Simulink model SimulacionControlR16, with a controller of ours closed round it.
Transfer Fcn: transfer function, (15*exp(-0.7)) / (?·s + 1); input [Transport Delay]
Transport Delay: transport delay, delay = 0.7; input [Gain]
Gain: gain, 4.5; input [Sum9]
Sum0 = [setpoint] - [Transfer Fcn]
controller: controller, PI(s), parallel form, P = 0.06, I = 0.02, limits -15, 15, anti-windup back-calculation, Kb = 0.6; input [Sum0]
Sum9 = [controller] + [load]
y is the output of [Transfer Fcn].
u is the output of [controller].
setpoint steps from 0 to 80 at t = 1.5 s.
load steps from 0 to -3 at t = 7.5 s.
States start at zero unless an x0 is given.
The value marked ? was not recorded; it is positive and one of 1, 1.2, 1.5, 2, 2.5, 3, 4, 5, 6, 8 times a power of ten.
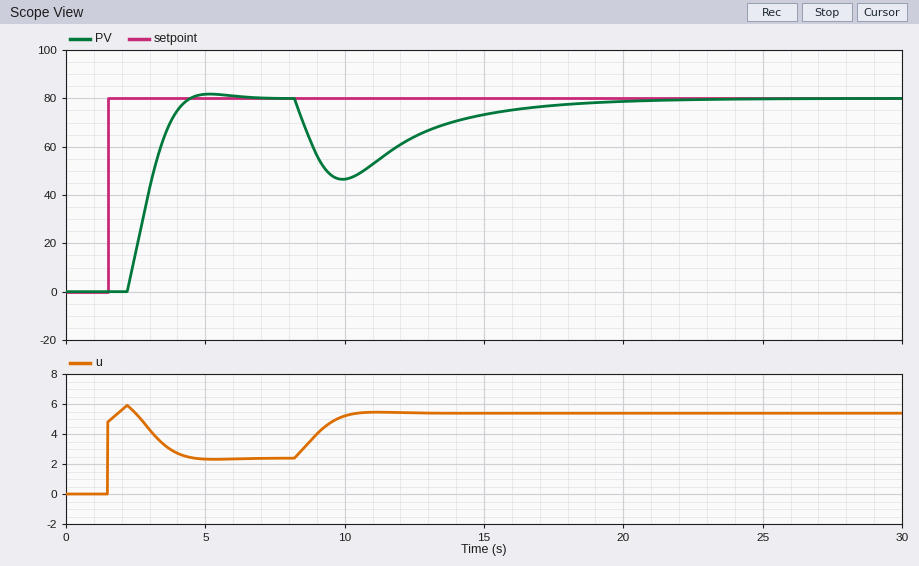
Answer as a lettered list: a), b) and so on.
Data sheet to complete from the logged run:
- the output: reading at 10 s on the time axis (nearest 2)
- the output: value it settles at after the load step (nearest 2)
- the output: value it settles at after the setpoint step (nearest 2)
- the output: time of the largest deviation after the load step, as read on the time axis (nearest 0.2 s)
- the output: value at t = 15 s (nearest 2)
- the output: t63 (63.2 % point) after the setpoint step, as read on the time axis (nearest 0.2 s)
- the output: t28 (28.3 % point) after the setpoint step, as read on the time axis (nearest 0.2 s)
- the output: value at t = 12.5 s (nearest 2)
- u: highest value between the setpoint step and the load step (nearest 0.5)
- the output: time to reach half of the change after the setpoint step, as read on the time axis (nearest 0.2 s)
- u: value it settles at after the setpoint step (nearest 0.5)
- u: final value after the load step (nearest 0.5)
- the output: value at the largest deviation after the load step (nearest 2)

a) 46
b) 80
c) 80
d) 10.0 s
e) 74
f) 3.2 s
g) 2.6 s
h) 64
i) 6.0
j) 3.0 s
k) 2.5
l) 5.5
m) 46
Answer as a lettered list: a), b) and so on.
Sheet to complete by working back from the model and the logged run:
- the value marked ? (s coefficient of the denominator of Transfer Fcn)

a) 3
